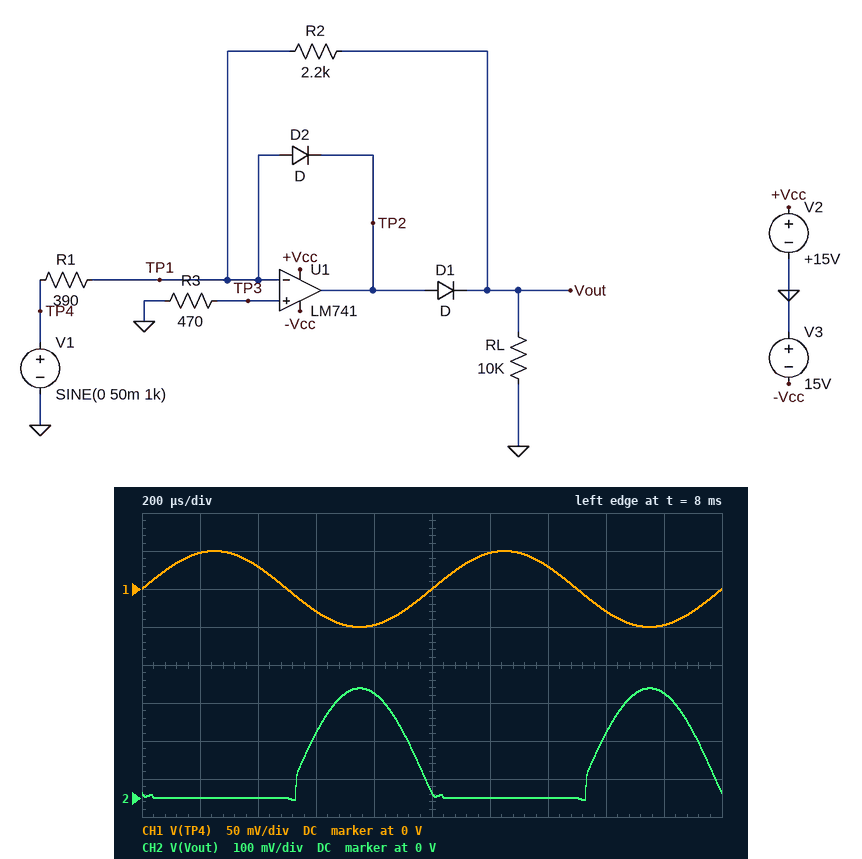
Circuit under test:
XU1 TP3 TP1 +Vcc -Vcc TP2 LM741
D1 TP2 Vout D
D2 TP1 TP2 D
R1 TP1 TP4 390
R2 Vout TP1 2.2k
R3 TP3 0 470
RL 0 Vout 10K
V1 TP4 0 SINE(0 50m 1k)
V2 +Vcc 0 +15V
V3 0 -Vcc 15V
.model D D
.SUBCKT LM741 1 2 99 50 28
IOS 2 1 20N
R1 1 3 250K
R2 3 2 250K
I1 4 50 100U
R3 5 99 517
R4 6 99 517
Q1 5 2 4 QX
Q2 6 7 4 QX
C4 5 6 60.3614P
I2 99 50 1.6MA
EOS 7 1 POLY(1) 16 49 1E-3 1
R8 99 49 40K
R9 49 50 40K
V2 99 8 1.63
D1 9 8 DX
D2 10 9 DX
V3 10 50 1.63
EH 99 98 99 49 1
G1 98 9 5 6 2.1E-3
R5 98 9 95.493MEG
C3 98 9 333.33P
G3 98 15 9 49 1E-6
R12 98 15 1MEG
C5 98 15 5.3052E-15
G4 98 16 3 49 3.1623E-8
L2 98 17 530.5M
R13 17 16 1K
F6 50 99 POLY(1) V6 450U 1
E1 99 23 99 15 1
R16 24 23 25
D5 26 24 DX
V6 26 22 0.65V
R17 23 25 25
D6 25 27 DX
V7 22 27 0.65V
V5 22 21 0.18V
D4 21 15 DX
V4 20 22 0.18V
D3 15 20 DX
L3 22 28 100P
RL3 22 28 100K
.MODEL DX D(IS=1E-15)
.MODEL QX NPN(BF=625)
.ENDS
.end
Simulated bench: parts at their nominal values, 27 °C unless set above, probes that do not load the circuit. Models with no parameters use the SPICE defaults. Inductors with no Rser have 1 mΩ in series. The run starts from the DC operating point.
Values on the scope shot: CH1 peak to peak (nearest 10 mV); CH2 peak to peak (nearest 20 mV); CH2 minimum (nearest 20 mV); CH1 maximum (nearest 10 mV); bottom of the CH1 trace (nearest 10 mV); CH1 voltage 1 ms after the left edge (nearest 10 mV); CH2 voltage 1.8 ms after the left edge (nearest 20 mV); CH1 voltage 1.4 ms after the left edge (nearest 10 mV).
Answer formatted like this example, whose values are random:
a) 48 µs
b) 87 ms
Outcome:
a) 100 mV
b) 300 mV
c) 0 V
d) 50 mV
e) -50 mV
f) 0 V
g) 280 mV
h) 30 mV
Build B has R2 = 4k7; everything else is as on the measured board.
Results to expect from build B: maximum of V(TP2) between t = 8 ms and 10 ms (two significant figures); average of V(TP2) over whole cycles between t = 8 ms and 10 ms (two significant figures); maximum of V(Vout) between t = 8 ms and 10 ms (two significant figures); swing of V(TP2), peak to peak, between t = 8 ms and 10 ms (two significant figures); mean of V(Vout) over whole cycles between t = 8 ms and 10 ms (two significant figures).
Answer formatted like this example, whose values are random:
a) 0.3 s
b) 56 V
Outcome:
a) 1.2 V
b) 210 mV
c) 620 mV
d) 1.8 V
e) 200 mV
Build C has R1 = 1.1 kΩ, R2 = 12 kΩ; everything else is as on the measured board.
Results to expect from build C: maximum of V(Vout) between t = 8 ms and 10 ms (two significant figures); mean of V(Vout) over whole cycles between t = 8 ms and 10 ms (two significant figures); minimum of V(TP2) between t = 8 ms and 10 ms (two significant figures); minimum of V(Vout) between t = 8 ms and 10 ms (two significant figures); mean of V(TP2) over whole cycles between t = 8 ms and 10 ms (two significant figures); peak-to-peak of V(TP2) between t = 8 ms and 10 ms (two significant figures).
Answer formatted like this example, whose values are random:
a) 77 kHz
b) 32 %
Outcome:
a) 560 mV
b) 180 mV
c) -570 mV
d) -3.5 mV
e) 200 mV
f) 1.7 V
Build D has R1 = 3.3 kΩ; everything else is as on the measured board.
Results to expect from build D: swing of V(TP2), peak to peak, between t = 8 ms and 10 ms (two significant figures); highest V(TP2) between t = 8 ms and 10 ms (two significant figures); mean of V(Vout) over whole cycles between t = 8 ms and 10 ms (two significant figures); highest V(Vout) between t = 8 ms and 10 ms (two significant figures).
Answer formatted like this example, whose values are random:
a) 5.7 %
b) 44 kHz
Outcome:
a) 1.1 V
b) 590 mV
c) 12 mV
d) 35 mV
